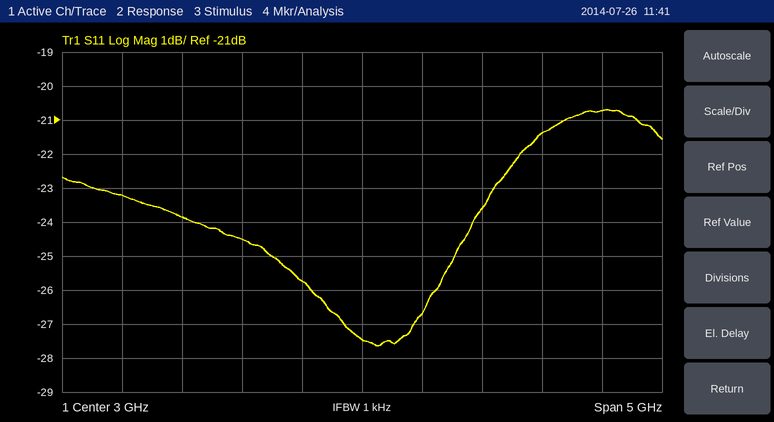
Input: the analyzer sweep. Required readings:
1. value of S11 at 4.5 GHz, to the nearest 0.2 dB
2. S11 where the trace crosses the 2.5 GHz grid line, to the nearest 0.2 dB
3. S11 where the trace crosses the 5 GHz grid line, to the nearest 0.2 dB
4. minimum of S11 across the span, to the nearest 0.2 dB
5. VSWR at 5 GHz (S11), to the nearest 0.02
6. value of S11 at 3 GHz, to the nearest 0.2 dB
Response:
-21.4 dB
-25.8 dB
-20.8 dB
-27.6 dB
1.20
-27.4 dB
